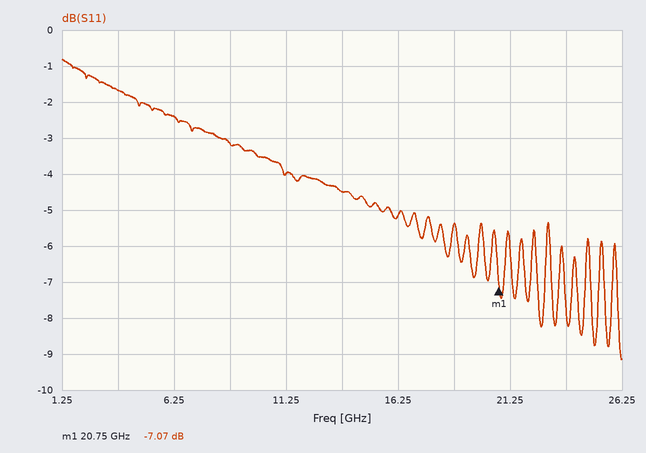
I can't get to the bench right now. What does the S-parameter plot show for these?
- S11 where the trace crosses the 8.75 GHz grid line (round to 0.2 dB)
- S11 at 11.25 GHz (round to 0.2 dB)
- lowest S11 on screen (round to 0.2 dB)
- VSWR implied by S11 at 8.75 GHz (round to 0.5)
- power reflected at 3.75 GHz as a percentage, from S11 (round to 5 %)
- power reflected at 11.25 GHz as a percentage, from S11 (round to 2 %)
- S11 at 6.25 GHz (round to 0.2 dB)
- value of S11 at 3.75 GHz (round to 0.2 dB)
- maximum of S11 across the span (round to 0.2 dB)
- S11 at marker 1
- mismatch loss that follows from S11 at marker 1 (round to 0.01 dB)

-3.2 dB
-4.0 dB
-9.2 dB
5.5
70 %
40 %
-2.4 dB
-1.6 dB
-0.8 dB
-7.07 dB
0.95 dB
